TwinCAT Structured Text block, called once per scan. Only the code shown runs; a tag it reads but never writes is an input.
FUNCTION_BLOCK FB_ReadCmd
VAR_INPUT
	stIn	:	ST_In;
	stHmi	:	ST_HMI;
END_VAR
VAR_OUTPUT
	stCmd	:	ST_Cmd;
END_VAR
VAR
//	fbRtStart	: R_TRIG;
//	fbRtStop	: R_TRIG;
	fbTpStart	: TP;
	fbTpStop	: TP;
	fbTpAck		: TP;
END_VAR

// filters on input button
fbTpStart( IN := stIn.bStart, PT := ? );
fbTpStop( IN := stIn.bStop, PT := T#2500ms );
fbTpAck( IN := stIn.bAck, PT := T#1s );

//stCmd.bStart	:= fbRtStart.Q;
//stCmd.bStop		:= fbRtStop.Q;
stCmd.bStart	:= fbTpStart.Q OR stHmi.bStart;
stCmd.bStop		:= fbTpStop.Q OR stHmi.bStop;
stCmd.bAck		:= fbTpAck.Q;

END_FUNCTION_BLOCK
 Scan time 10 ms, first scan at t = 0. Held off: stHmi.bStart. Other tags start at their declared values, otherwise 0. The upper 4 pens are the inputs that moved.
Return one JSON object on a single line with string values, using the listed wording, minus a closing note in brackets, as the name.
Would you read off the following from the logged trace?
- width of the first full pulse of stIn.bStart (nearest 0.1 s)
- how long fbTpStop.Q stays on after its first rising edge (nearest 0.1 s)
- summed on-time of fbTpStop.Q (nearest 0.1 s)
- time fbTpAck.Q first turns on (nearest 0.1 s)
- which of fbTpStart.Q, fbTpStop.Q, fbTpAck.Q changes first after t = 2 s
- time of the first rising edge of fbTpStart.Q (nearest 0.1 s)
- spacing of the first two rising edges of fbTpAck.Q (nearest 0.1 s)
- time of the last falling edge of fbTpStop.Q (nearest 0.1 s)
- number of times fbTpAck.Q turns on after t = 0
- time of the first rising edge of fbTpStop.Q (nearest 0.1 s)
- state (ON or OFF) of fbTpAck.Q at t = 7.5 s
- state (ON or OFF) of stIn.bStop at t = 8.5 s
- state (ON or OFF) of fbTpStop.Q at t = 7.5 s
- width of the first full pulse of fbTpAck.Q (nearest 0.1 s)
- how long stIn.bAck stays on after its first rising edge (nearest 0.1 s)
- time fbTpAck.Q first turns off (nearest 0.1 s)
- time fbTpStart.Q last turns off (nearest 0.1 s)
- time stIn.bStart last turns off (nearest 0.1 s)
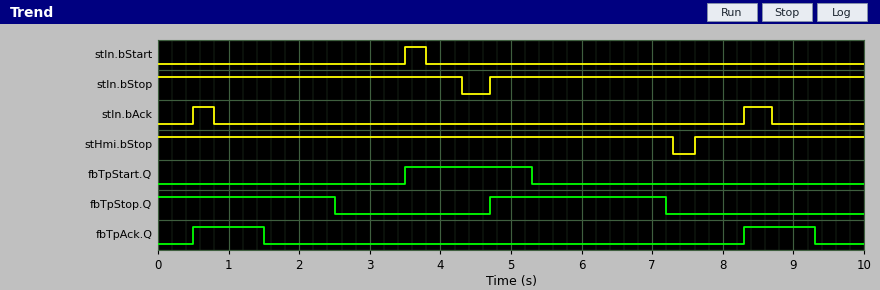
{"width of the first full pulse of stIn.bStart": "0.3 s", "how long fbTpStop.Q stays on after its first rising edge": "2.5 s", "summed on-time of fbTpStop.Q": "5.0 s", "time fbTpAck.Q first turns on": "0.5 s", "which of fbTpStart.Q, fbTpStop.Q, fbTpAck.Q changes first after t = 2 s": "fbTpStop.Q", "time of the first rising edge of fbTpStart.Q": "3.5 s", "spacing of the first two rising edges of fbTpAck.Q": "7.8 s", "time of the last falling edge of fbTpStop.Q": "7.2 s", "number of times fbTpAck.Q turns on after t = 0": "2", "time of the first rising edge of fbTpStop.Q": "4.7 s", "state (ON or OFF) of fbTpAck.Q at t = 7.5 s": "OFF", "state (ON or OFF) of stIn.bStop at t = 8.5 s": "ON", "state (ON or OFF) of fbTpStop.Q at t = 7.5 s": "OFF", "width of the first full pulse of fbTpAck.Q": "1.0 s", "how long stIn.bAck stays on after its first rising edge": "0.3 s", "time fbTpAck.Q first turns off": "1.5 s", "time fbTpStart.Q last turns off": "5.3 s", "time stIn.bStart last turns off": "3.8 s"}
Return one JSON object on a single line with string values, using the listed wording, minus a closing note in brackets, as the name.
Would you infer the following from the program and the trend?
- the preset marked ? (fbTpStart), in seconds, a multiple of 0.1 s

{"the preset marked ? (fbTpStart), in seconds, a multiple of 0.1 s": "1.8 s"}
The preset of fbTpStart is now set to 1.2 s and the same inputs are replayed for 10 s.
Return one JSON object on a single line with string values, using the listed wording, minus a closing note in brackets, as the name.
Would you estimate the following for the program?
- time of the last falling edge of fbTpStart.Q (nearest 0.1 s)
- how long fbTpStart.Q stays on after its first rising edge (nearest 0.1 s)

{"time of the last falling edge of fbTpStart.Q": "4.7 s", "how long fbTpStart.Q stays on after its first rising edge": "1.2 s"}
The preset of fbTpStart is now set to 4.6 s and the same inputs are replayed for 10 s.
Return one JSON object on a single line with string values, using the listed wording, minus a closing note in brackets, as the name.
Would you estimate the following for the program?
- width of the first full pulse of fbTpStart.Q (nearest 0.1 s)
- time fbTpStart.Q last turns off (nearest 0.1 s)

{"width of the first full pulse of fbTpStart.Q": "4.6 s", "time fbTpStart.Q last turns off": "8.1 s"}
